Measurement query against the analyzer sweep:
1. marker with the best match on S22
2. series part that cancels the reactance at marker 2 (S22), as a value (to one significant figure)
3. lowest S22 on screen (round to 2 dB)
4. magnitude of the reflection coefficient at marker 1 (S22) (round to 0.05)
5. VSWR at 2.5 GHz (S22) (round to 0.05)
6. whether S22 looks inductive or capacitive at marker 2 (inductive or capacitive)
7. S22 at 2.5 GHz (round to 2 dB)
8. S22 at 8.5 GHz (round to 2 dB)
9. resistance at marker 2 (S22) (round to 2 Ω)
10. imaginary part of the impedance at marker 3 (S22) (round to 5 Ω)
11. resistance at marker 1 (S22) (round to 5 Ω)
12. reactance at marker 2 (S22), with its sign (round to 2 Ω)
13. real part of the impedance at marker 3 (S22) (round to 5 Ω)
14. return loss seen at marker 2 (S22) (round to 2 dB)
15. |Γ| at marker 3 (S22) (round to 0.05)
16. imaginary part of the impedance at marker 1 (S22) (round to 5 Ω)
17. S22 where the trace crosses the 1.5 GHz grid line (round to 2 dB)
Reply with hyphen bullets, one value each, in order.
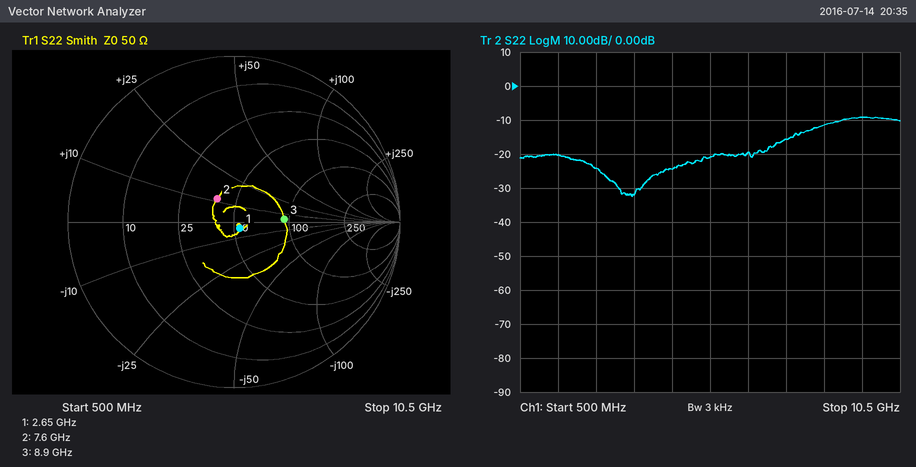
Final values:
- marker 1
- 2 pF
- -32 dB
- 0.05
- 1.15
- inductive
- -24 dB
- -12 dB
- 40 Ω
- +5 Ω
- 55 Ω
- +12 Ω
- 95 Ω
- 16 dB
- 0.30
- -5 Ω
- -20 dB
